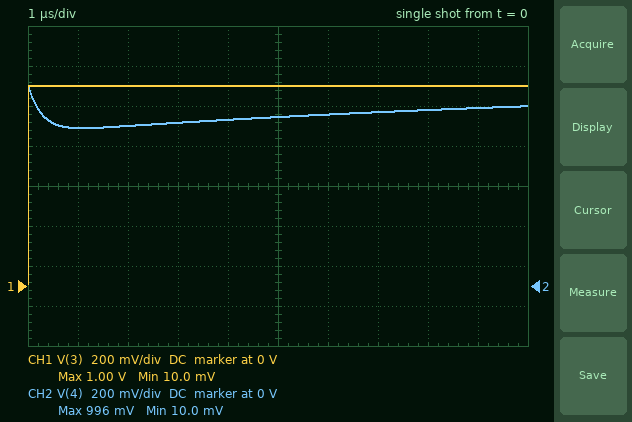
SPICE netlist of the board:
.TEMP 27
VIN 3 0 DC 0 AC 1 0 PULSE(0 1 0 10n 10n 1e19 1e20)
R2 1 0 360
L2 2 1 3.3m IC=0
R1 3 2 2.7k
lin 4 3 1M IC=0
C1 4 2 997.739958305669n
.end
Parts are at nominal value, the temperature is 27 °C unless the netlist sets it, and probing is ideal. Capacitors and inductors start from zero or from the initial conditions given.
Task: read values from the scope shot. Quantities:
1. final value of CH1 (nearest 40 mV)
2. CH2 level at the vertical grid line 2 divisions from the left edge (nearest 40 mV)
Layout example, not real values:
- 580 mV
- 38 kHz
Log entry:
- 1.00 V
- 800 mV
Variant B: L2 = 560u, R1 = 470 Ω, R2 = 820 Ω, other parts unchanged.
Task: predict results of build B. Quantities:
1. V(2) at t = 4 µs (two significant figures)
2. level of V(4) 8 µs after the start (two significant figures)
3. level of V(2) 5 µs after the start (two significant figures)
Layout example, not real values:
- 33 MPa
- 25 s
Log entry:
- 870 mV
- 960 mV
- 900 mV
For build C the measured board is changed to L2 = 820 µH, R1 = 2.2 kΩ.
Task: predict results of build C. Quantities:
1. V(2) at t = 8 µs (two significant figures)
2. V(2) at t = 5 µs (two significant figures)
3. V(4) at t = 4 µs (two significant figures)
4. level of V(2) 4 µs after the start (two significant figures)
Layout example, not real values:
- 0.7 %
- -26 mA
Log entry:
- 870 mV
- 790 mV
- 750 mV
- 740 mV
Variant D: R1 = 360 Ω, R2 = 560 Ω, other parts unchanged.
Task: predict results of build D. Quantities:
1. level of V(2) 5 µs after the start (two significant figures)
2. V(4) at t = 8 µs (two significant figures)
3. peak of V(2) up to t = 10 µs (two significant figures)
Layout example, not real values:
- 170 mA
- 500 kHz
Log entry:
- 870 mV
- 900 mV
- 1.0 V
